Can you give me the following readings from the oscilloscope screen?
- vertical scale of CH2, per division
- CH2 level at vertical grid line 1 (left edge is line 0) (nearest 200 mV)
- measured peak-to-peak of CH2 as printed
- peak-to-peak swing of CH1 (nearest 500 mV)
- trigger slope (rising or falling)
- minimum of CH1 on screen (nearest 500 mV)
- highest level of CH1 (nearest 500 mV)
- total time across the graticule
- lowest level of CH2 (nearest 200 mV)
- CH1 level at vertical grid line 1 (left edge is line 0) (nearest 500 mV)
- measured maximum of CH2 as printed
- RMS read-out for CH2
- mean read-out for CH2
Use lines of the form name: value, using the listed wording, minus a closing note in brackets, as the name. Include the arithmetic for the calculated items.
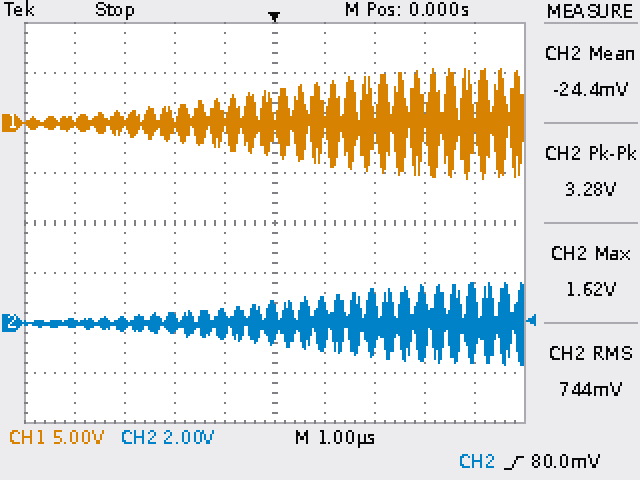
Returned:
vertical scale of CH2, per division: 2 V
CH2 level at vertical grid line 1 (left edge is line 0): 0.0 V
measured peak-to-peak of CH2 as printed: 3.28 V
peak-to-peak swing of CH1: 5.5 V − (-5.5 V) = 11.0 V
trigger slope: rising
minimum of CH1 on screen: -5.5 V
highest level of CH1: 5.5 V
total time across the graticule: 10 µs
lowest level of CH2: -1.6 V
CH1 level at vertical grid line 1 (left edge is line 0): 0.0 V
measured maximum of CH2 as printed: 1.62 V
RMS read-out for CH2: 744 mV
mean read-out for CH2: -24.4 mV
